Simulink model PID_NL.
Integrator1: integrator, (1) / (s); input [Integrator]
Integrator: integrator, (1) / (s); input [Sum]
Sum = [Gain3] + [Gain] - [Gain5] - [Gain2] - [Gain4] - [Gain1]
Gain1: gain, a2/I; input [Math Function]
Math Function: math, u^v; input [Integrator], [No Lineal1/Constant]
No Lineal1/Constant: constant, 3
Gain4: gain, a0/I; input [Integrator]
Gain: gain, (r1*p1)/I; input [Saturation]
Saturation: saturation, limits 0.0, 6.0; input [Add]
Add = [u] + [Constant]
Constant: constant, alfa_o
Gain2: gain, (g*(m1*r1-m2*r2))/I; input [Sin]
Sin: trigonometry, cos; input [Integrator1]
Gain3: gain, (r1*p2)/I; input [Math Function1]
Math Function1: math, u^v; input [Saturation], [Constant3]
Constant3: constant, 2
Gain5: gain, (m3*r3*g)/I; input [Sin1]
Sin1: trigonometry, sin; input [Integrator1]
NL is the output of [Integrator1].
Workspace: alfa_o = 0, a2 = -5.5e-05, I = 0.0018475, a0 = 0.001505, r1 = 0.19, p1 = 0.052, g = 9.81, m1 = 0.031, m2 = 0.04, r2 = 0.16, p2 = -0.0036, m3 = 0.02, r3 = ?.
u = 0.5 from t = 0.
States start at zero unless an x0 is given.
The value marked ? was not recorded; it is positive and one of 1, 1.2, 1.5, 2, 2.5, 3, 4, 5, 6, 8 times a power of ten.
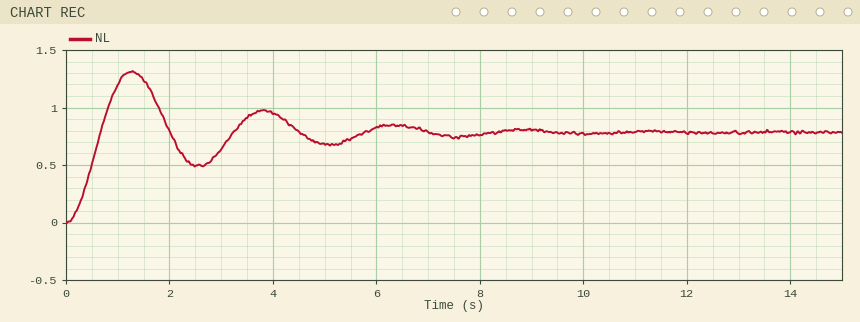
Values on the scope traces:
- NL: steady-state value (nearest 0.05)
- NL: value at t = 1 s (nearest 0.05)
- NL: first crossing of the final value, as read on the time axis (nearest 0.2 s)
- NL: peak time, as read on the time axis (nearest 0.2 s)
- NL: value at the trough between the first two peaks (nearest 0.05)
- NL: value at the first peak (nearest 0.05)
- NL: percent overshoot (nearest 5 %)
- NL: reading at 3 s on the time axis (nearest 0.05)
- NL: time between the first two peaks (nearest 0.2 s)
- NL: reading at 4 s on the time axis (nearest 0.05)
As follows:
0.80
1.20
0.6 s
1.2 s
0.50
1.30
65 %
0.65
2.6 s
0.95
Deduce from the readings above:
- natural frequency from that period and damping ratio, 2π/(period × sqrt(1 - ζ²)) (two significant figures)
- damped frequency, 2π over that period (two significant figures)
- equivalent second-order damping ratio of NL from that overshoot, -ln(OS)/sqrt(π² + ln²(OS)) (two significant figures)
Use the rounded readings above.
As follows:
2.4 rad/s
2.4 rad/s
0.14
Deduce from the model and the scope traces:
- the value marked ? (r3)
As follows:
0.06
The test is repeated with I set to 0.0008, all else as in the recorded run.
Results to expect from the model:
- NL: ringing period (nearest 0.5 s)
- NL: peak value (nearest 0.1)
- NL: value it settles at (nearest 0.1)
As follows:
1.5 s
1.2
0.8
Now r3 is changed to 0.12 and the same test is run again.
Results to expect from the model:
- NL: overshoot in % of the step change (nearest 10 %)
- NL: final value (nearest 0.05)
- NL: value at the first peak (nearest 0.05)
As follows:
70 %
0.40
0.70
